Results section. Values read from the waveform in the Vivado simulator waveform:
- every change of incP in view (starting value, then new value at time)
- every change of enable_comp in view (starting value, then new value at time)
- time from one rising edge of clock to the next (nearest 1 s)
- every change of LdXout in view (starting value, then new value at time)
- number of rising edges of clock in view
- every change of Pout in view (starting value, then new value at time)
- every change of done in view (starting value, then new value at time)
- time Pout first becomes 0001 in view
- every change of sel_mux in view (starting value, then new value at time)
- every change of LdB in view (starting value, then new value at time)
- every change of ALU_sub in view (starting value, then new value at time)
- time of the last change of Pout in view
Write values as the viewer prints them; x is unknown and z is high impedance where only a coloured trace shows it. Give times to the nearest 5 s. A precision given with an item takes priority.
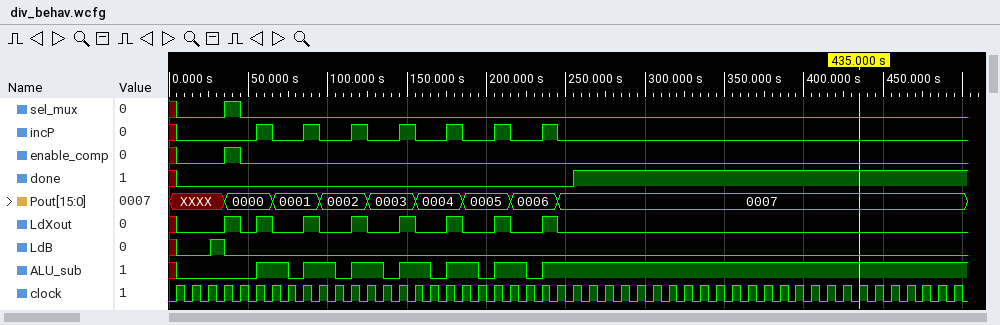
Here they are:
x, 0 at 5 s, 1 at 55 s, 0 at 65 s, 1 at 85 s, 0 at 95 s, 1 at 115 s, 0 at 125 s, 1 at 145 s, 0 at 155 s, 1 at 175 s, 0 at 185 s, 1 at 205 s, 0 at 215 s, 1 at 235 s, 0 at 245 s
x, 0 at 5 s, 1 at 35 s, 0 at 45 s
10 s
x, 0 at 5 s, 1 at 35 s, 0 at 45 s, 1 at 55 s, 0 at 65 s, 1 at 85 s, 0 at 95 s, 1 at 115 s, 0 at 125 s, 1 at 145 s, 0 at 155 s, 1 at 175 s, 0 at 185 s, 1 at 205 s, 0 at 215 s, 1 at 235 s, 0 at 245 s
50
XXXX, 0000 at 35 s, 0001 at 65 s, 0002 at 95 s, 0003 at 125 s, 0004 at 155 s, 0005 at 185 s, 0006 at 215 s, 0007 at 245 s
x, 0 at 5 s, 1 at 255 s
65 s
x, 0 at 5 s, 1 at 35 s, 0 at 45 s
x, 0 at 5 s, 1 at 25 s, 0 at 35 s
x, 0 at 5 s, 1 at 55 s, 0 at 75 s, 1 at 85 s, 0 at 105 s, 1 at 115 s, 0 at 135 s, 1 at 145 s, 0 at 165 s, 1 at 175 s, 0 at 195 s, 1 at 205 s, 0 at 225 s, 1 at 235 s
245 s
